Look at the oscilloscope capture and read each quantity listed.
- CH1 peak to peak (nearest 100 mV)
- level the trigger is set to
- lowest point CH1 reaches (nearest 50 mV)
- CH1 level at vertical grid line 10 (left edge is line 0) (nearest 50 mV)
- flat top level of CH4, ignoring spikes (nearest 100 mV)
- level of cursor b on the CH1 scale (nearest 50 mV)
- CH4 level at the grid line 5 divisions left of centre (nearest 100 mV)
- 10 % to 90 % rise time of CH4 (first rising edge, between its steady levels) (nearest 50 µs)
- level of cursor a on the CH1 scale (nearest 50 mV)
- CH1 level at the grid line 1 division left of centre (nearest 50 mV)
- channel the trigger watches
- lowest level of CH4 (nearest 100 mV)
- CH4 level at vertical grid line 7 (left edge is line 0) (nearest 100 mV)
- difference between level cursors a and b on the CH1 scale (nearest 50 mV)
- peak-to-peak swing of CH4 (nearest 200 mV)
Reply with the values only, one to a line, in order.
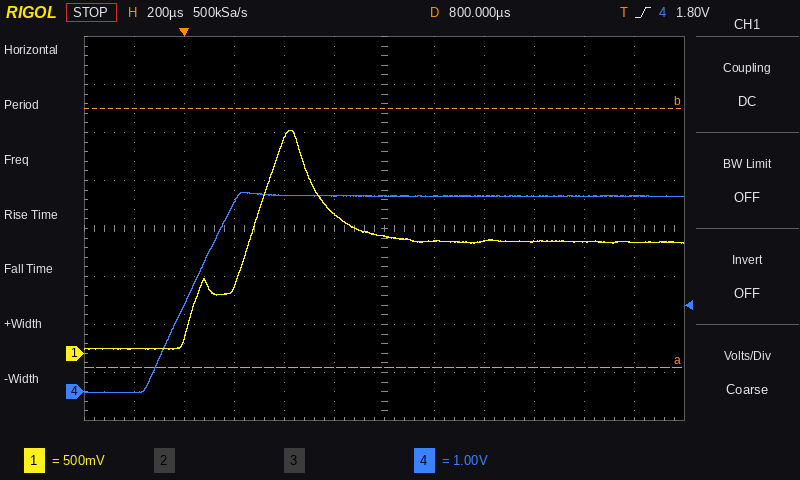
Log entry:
2.30 V
1.80 V
50 mV
1.15 V
4.1 V
2.55 V
0.0 V
300 µs
-150 mV
1.45 V
CH4
0.0 V
4.1 V
2.70 V
4.2 V
